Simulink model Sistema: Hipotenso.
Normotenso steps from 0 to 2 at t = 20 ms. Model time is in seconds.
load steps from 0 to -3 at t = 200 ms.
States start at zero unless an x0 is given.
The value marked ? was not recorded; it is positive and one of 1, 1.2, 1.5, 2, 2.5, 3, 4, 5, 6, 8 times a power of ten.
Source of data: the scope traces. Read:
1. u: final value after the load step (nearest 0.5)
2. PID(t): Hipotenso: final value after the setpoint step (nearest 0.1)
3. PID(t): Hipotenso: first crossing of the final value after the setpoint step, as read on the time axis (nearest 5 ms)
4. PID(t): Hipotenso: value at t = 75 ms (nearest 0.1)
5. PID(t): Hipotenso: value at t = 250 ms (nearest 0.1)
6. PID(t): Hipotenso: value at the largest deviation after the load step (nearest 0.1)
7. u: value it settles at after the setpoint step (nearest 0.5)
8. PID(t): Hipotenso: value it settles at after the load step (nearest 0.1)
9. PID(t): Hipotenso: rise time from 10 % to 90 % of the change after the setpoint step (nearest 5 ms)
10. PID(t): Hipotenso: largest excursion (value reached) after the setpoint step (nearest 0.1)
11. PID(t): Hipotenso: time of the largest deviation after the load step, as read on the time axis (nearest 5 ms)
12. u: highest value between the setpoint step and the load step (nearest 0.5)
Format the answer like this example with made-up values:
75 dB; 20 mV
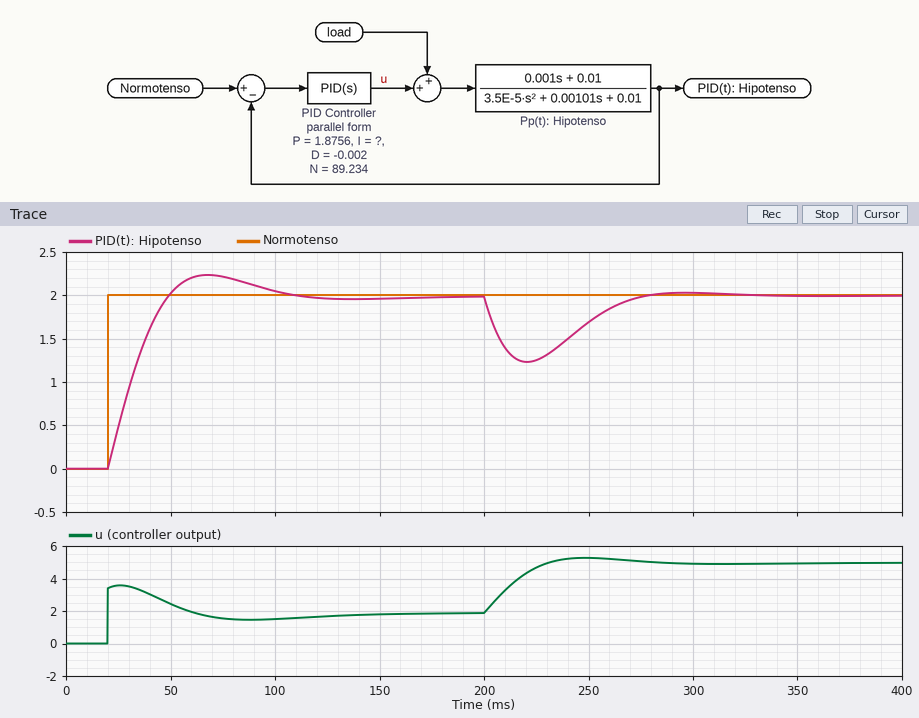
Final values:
5.0; 2.0; 50 ms; 2.2; 1.7; 1.2; 2.0; 2.0; 20 ms; 2.2; 220 ms; 3.5
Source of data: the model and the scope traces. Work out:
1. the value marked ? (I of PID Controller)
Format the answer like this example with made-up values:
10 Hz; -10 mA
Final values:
100
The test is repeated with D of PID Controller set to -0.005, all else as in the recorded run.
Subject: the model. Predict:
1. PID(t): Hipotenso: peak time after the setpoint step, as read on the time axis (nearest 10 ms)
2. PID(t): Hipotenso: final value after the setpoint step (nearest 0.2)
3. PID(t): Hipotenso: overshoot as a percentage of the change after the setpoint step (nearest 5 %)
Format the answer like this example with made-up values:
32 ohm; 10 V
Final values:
70 ms; 2.0; 15 %
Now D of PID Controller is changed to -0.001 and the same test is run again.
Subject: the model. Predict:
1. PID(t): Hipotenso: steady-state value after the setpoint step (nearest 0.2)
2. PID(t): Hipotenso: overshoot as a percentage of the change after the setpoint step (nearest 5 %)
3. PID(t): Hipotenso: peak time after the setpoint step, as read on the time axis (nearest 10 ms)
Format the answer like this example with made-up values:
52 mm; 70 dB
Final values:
2.0; 10 %; 70 ms
